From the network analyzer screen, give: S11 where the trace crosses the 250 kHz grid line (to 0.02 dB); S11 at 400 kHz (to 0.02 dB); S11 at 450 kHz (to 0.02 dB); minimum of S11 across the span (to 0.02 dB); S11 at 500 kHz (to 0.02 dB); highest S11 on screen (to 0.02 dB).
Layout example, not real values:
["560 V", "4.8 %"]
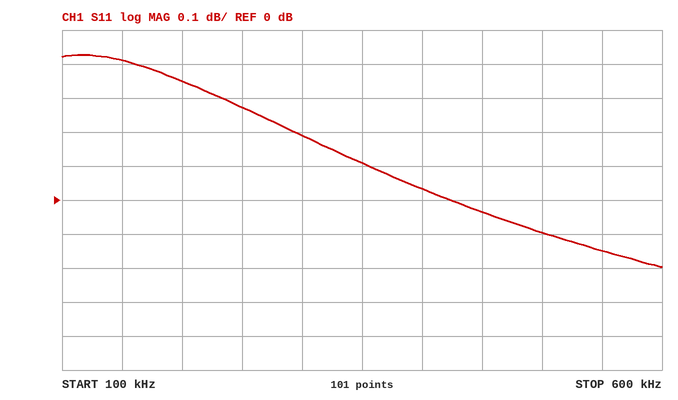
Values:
["0.28 dB", "0.04 dB", "-0.04 dB", "-0.20 dB", "-0.10 dB", "0.42 dB"]
